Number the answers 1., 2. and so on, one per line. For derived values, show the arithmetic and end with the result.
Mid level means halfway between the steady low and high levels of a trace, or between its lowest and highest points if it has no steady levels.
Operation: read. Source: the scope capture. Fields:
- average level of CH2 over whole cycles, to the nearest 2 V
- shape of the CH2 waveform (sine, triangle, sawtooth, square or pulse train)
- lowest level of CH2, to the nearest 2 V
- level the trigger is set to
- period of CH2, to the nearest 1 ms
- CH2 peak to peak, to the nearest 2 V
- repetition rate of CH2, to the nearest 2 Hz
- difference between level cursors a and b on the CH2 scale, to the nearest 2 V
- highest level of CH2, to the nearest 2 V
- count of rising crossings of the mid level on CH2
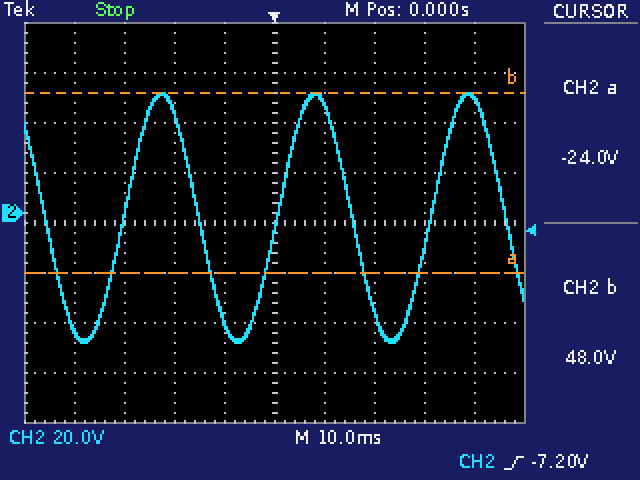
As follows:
1. (48 V + (-52 V)) / 2 ≈ -2 V
2. sine
3. -52 V
4. -7.20 V
5. 31 ms
6. 48 V − (-52 V) = 100 V
7. 1 / 31 ms ≈ 32 Hz
8. 72 V
9. 48 V
10. 3
